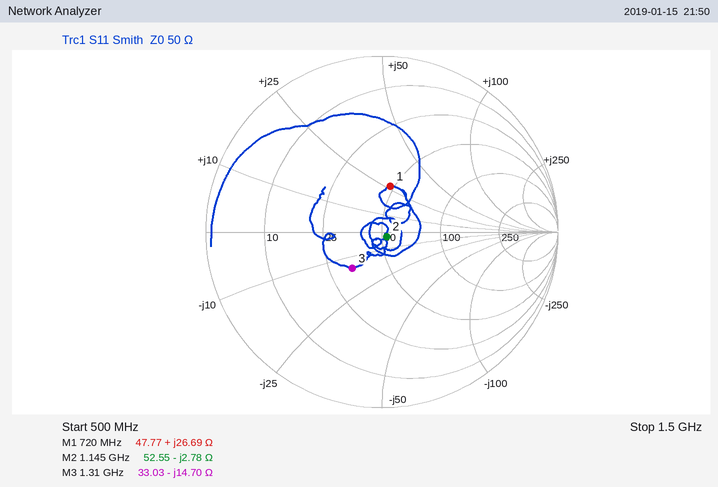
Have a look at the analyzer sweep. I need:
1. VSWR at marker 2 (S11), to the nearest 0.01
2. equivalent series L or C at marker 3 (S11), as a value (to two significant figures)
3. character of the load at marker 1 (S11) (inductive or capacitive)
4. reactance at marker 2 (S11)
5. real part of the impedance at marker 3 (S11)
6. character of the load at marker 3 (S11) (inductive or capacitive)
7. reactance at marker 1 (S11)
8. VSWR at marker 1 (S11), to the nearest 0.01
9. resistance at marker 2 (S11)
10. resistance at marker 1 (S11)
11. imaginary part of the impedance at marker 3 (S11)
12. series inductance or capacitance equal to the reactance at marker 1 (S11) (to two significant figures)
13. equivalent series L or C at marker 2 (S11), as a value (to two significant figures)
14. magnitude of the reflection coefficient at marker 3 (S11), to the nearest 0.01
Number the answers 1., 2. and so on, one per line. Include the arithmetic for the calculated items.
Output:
1. 1.08
2. C = 1/(2π × 1.31 GHz × 14.7 Ω) ≈ 8.3 pF
3. inductive
4. -2.78 Ω
5. 33.03 Ω
6. capacitive
7. +26.69 Ω
8. 1.72
9. 52.55 Ω
10. 47.77 Ω
11. -14.70 Ω
12. L = 26.69 Ω/(2π × 720 MHz) ≈ 5.9 nH
13. C = 1/(2π × 1.145 GHz × 2.78 Ω) ≈ 50 pF
14. 0.27
